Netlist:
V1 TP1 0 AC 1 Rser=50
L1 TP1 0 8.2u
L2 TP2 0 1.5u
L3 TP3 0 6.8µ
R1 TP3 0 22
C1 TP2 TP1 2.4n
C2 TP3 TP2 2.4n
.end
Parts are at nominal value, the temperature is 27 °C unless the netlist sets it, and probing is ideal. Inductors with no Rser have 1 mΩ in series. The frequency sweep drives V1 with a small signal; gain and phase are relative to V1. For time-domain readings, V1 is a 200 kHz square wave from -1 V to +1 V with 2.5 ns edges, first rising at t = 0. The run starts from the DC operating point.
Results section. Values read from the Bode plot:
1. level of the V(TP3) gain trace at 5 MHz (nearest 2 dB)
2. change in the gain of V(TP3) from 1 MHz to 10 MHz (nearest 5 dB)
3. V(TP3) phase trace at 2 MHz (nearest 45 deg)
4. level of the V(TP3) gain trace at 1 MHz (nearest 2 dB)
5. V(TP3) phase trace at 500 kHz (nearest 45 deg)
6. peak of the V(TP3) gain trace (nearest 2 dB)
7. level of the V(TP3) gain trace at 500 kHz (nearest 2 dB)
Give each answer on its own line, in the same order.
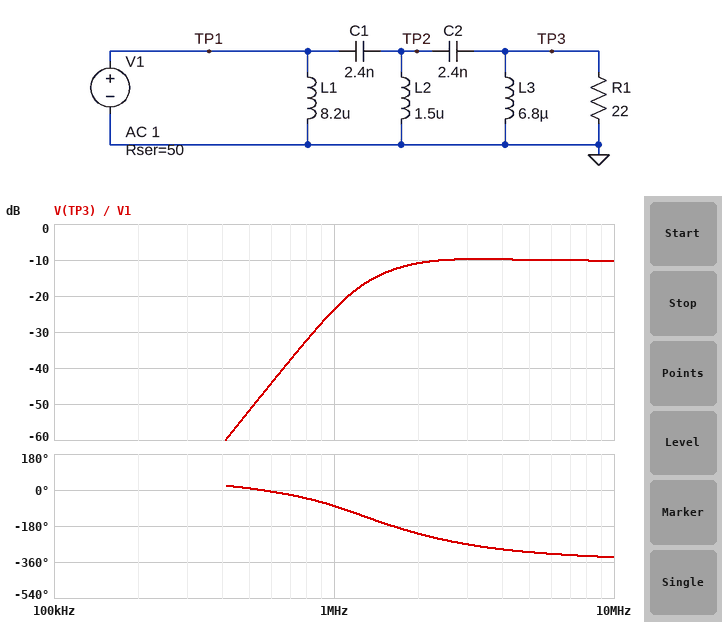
-10 dB
15 dB
-225 deg
-24 dB
0 deg
-10 dB
-52 dB
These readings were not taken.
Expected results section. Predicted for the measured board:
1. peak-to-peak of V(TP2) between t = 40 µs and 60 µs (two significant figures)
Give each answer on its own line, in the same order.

1.2 V
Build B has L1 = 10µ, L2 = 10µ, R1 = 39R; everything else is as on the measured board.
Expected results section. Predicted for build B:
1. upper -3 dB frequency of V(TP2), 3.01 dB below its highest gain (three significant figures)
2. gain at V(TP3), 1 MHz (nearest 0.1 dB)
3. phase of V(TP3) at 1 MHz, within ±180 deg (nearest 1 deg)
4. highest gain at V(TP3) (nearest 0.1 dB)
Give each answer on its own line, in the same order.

722 kHz
-9.8 dB
159 deg
-7.2 dB
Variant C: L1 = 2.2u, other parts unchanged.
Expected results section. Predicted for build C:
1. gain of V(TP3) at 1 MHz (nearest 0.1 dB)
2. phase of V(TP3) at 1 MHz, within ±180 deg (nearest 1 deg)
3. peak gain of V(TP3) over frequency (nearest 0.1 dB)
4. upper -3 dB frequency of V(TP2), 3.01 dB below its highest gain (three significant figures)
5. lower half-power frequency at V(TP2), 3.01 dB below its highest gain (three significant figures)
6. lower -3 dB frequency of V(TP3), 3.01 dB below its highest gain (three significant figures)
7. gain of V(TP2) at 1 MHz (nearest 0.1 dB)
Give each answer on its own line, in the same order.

-32.9 dB
-14 deg
-9.7 dB
2.23 MHz
1.43 MHz
1.46 MHz
-23.2 dB
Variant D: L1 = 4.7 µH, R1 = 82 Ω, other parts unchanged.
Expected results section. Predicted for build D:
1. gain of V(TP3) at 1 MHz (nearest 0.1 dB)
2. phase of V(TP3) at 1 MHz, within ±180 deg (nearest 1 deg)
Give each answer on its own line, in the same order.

-15.2 dB
-29 deg
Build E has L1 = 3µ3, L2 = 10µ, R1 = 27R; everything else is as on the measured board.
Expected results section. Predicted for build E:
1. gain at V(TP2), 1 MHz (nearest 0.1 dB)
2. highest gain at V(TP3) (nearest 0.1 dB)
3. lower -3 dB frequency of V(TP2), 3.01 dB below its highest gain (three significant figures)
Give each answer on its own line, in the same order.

-9.2 dB
-8.8 dB
649 kHz
